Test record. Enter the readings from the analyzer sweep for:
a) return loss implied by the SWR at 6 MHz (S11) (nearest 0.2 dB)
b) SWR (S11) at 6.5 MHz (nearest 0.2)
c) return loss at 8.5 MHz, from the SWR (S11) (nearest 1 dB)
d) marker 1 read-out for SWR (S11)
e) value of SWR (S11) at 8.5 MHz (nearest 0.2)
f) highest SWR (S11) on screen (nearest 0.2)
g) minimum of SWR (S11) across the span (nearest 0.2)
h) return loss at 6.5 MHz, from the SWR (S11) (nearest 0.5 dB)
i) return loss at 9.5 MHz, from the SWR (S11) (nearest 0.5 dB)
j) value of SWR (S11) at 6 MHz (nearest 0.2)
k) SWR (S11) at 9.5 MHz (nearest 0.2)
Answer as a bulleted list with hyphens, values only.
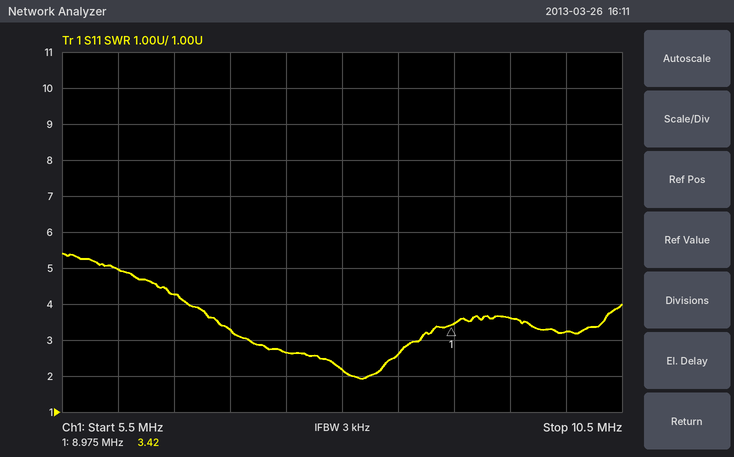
- 3.6 dB
- 4.2
- 7 dB
- 3.42
- 2.6
- 5.4
- 2.0
- 4.0 dB
- 5.0 dB
- 5.0
- 3.6
